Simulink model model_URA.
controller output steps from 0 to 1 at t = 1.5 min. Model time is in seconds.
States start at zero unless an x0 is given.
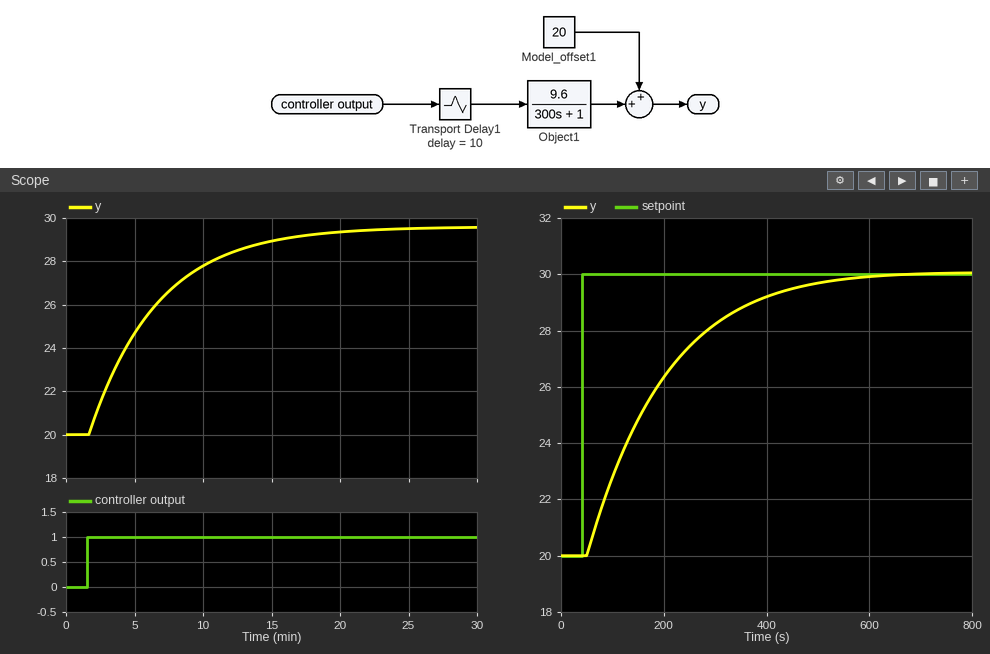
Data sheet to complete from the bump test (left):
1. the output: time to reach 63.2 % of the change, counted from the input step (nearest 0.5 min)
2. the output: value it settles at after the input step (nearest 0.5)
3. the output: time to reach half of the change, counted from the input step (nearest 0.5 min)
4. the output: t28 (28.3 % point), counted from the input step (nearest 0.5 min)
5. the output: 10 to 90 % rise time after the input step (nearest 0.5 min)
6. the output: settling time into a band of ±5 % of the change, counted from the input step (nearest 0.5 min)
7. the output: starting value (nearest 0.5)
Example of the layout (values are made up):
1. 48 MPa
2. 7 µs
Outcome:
1. 5.0 min
2. 29.5
3. 3.5 min
4. 2.0 min
5. 11.0 min
6. 15.0 min
7. 20.0
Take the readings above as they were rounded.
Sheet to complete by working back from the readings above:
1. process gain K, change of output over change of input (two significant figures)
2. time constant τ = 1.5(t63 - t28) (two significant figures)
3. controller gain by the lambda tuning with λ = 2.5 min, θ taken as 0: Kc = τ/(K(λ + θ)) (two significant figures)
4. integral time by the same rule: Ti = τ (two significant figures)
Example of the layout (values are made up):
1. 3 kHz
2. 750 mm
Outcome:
1. 9.5
2. 4.5 min
3. 0.19
4. 4.5 min
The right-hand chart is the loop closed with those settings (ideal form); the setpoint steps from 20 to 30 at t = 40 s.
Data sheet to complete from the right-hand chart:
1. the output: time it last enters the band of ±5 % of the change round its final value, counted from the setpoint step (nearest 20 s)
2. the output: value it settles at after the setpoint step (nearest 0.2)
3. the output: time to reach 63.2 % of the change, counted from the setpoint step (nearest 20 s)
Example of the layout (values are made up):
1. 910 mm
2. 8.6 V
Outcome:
1. 420 s
2. 30.0
3. 160 s
